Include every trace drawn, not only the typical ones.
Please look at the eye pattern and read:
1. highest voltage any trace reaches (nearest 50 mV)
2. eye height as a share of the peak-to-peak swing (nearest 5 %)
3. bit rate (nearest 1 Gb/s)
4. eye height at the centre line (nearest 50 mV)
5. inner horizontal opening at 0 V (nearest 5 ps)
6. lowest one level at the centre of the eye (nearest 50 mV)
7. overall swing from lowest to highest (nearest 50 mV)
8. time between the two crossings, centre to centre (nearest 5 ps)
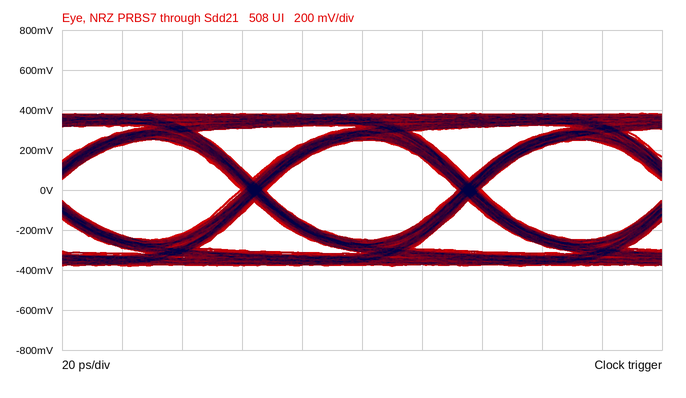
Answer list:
400 mV
65 %
14 Gb/s
500 mV
65 ps
250 mV
750 mV
70 ps
